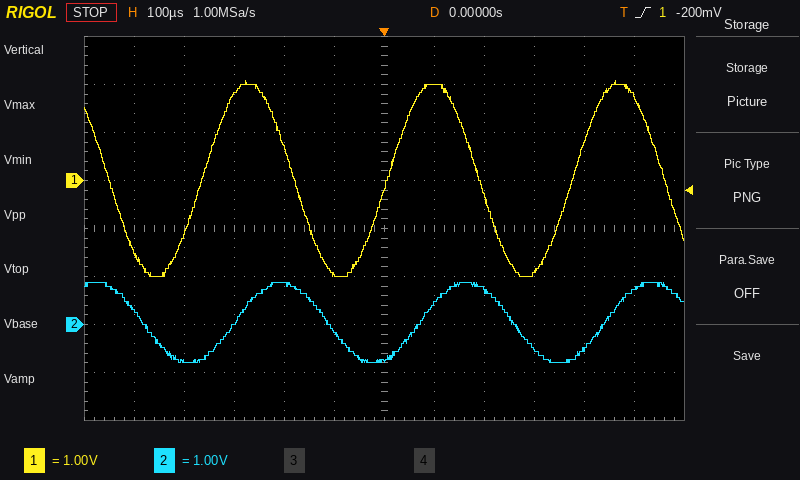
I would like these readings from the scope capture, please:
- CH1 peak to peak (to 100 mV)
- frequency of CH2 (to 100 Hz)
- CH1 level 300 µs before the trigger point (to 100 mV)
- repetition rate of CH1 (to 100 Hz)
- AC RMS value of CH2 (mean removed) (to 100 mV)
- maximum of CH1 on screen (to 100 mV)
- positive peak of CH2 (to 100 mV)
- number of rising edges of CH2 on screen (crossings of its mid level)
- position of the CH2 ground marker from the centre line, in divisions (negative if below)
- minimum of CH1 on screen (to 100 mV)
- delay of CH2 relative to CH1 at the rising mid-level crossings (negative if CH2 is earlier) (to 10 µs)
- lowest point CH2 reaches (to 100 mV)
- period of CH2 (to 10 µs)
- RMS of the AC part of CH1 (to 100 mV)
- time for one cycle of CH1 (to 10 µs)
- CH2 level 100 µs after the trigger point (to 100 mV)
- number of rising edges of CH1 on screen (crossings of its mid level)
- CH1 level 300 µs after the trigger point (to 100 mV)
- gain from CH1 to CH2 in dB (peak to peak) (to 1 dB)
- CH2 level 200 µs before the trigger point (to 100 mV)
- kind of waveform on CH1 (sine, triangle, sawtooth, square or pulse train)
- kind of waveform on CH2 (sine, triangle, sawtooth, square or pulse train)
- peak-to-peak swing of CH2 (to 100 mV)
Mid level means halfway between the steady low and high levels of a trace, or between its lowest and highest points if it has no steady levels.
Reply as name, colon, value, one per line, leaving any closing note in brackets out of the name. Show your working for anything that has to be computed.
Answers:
CH1 peak to peak: 2.1 V − (-2.0 V) = 4.1 V
frequency of CH2: 1 / 370 µs ≈ 2.7 kHz
CH1 level 300 µs before the trigger point: 1.8 V
repetition rate of CH1: 1 / 370 µs ≈ 2.7 kHz
AC RMS value of CH2 (mean removed): 1.7 V / (2√2) ≈ 601 mV, so 600 mV to the nearest 100 mV
maximum of CH1 on screen: 2.1 V
positive peak of CH2: 900 mV
number of rising edges of CH2 on screen: 3
position of the CH2 ground marker from the centre line, in divisions: -2.0 div
minimum of CH1 on screen: -2.0 V
delay of CH2 relative to CH1 at the rising mid-level crossings (negative if CH2 is earlier): +70 µs
lowest point CH2 reaches: -800 mV
period of CH2: 370 µs
RMS of the AC part of CH1: 4.1 V / (2√2) ≈ 1.4 V
time for one cycle of CH1: 370 µs
CH2 level 100 µs after the trigger point: 400 mV
number of rising edges of CH1 on screen: 3
CH1 level 300 µs after the trigger point: -1.9 V
gain from CH1 to CH2 in dB (peak to peak): 20 log10(1.7 V / 4.1 V) ≈ -8 dB
CH2 level 200 µs before the trigger point: 800 mV
kind of waveform on CH1: sine
kind of waveform on CH2: sine
peak-to-peak swing of CH2: 900 mV − (-800 mV) = 1.7 V
